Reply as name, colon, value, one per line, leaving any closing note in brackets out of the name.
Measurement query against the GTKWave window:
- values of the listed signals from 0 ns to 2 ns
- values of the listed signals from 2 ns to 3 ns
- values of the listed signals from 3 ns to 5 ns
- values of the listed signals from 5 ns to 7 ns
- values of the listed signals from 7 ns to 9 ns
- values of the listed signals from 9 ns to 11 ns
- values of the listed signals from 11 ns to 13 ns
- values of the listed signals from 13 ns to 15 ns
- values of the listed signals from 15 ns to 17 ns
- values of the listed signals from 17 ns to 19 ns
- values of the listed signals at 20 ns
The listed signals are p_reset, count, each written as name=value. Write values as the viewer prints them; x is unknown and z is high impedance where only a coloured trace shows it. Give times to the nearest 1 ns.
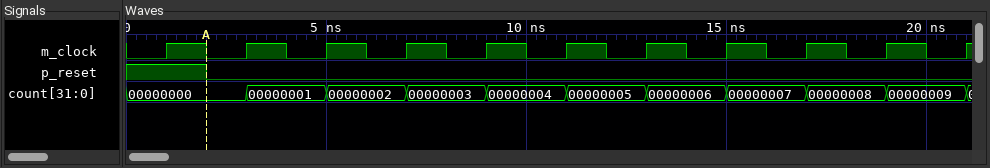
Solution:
values of the listed signals from 0 ns to 2 ns: p_reset=1, count=00000000
values of the listed signals from 2 ns to 3 ns: p_reset=0, count=00000000
values of the listed signals from 3 ns to 5 ns: p_reset=0, count=00000001
values of the listed signals from 5 ns to 7 ns: p_reset=0, count=00000002
values of the listed signals from 7 ns to 9 ns: p_reset=0, count=00000003
values of the listed signals from 9 ns to 11 ns: p_reset=0, count=00000004
values of the listed signals from 11 ns to 13 ns: p_reset=0, count=00000005
values of the listed signals from 13 ns to 15 ns: p_reset=0, count=00000006
values of the listed signals from 15 ns to 17 ns: p_reset=0, count=00000007
values of the listed signals from 17 ns to 19 ns: p_reset=0, count=00000008
values of the listed signals at 20 ns: p_reset=0, count=00000009
